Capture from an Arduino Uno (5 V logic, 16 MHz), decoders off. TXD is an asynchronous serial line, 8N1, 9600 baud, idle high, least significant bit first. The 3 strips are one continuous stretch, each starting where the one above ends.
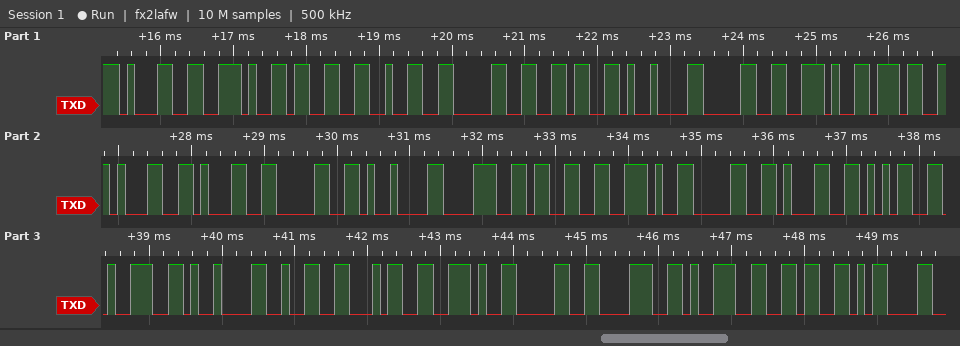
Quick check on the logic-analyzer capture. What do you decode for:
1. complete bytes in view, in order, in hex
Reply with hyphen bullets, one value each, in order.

- 31 2E 33 32 30 36 09 30 2E 37 31 31 30 09 38 33 2E 30 31 35 39 09 32 34 2E 30 38 39 36 0D
